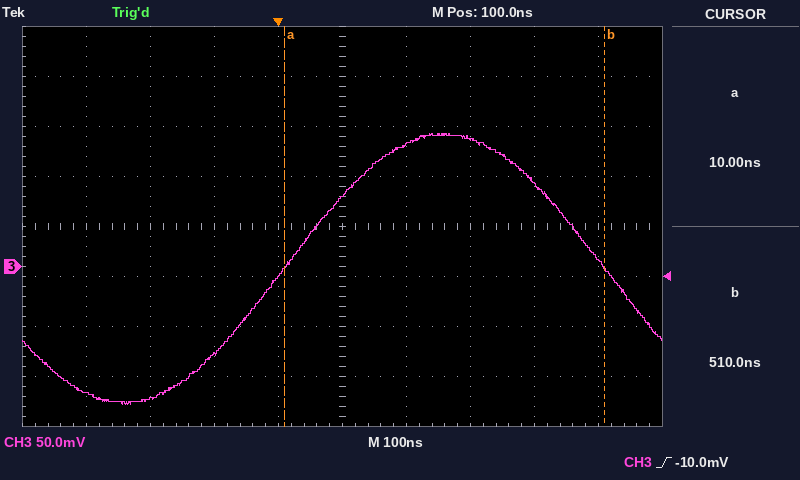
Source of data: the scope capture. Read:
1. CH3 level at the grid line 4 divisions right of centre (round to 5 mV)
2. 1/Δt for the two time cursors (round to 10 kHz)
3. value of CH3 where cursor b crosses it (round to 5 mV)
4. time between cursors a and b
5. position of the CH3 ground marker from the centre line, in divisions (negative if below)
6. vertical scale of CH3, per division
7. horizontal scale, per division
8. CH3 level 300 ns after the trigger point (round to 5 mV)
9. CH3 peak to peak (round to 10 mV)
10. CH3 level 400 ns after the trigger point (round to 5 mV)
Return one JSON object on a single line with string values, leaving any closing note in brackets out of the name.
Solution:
{"CH3 level at the grid line 4 divisions right of centre": "10 mV", "1/Δt for the two time cursors": "2.00 MHz", "value of CH3 where cursor b crosses it": "0 mV", "time between cursors a and b": "500 ns", "position of the CH3 ground marker from the centre line, in divisions": "-0.8 div", "vertical scale of CH3, per division": "50 mV", "horizontal scale, per division": "100 ns", "CH3 level 300 ns after the trigger point": "130 mV", "CH3 peak to peak": "270 mV", "CH3 level 400 ns after the trigger point": "85 mV"}
